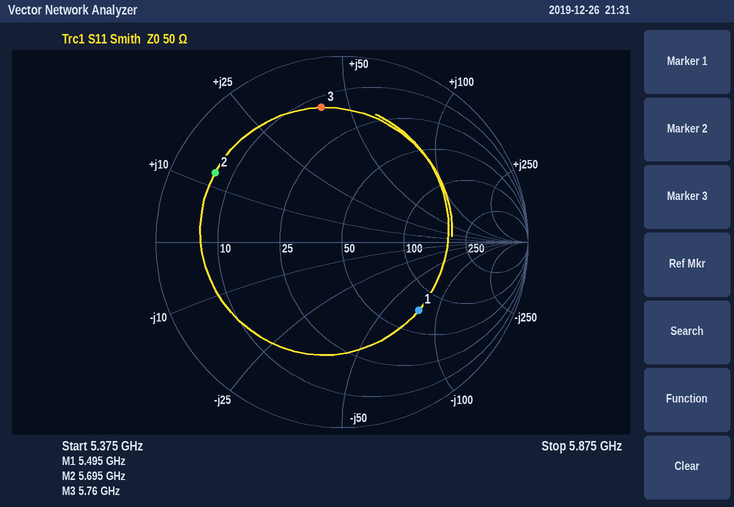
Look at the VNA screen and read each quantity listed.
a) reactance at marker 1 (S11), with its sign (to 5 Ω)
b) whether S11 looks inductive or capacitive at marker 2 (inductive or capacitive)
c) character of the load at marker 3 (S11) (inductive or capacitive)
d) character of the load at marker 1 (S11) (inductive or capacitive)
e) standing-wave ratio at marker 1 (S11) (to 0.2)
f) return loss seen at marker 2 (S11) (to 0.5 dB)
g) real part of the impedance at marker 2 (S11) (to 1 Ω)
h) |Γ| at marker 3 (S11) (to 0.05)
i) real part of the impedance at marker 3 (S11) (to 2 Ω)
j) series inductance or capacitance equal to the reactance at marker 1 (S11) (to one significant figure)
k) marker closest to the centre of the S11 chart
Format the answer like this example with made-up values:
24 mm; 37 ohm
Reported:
-75 Ω; inductive; inductive; capacitive; 3.4; 2.0 dB; 7 Ω; 0.75; 14 Ω; 400 fF; marker 1
